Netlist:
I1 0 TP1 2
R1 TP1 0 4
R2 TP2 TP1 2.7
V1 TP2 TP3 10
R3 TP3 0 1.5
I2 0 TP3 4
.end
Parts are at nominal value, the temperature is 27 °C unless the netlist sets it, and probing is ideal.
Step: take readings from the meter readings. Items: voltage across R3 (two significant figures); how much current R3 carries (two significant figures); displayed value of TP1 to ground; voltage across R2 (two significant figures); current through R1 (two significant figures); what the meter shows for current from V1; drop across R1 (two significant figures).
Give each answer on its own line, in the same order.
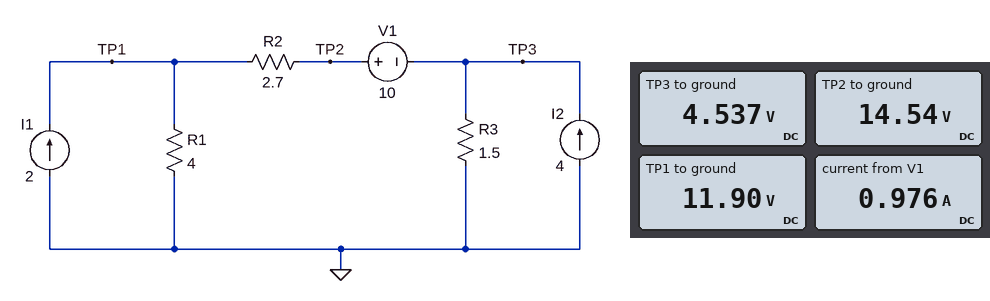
4.5 V
3.0 A
11.90 V
2.6 V
3.0 A
0.976 A
12 V
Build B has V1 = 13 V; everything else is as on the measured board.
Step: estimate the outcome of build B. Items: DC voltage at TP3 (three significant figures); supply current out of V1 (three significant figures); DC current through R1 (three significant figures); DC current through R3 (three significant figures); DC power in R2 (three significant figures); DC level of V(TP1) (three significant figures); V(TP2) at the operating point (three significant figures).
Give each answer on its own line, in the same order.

3.99 V
1.34 A
3.34 A
2.66 A
4.86 W
13.4 V
17.0 V
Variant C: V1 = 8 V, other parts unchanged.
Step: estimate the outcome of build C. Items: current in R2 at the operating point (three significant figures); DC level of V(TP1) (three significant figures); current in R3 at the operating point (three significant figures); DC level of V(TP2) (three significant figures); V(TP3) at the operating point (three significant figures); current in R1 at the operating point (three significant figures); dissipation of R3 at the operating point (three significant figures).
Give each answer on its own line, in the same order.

732 mA
10.9 V
3.27 A
12.9 V
4.90 V
2.73 A
16.0 W
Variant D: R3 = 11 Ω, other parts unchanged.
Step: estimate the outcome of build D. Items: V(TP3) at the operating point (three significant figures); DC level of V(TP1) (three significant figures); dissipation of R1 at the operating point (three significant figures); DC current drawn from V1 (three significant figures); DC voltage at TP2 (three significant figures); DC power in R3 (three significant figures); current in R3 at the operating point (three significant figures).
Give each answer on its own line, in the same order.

15.4 V
18.4 V
84.6 W
2.60 A
25.4 V
21.6 W
1.40 A
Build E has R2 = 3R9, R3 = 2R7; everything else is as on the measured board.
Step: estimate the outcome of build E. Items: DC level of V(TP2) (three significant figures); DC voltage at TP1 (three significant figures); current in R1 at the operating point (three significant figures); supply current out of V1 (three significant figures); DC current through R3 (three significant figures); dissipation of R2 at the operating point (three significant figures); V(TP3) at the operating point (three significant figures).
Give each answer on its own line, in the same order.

17.5 V
12.8 V
3.21 A
1.21 A
2.79 A
5.69 W
7.54 V
